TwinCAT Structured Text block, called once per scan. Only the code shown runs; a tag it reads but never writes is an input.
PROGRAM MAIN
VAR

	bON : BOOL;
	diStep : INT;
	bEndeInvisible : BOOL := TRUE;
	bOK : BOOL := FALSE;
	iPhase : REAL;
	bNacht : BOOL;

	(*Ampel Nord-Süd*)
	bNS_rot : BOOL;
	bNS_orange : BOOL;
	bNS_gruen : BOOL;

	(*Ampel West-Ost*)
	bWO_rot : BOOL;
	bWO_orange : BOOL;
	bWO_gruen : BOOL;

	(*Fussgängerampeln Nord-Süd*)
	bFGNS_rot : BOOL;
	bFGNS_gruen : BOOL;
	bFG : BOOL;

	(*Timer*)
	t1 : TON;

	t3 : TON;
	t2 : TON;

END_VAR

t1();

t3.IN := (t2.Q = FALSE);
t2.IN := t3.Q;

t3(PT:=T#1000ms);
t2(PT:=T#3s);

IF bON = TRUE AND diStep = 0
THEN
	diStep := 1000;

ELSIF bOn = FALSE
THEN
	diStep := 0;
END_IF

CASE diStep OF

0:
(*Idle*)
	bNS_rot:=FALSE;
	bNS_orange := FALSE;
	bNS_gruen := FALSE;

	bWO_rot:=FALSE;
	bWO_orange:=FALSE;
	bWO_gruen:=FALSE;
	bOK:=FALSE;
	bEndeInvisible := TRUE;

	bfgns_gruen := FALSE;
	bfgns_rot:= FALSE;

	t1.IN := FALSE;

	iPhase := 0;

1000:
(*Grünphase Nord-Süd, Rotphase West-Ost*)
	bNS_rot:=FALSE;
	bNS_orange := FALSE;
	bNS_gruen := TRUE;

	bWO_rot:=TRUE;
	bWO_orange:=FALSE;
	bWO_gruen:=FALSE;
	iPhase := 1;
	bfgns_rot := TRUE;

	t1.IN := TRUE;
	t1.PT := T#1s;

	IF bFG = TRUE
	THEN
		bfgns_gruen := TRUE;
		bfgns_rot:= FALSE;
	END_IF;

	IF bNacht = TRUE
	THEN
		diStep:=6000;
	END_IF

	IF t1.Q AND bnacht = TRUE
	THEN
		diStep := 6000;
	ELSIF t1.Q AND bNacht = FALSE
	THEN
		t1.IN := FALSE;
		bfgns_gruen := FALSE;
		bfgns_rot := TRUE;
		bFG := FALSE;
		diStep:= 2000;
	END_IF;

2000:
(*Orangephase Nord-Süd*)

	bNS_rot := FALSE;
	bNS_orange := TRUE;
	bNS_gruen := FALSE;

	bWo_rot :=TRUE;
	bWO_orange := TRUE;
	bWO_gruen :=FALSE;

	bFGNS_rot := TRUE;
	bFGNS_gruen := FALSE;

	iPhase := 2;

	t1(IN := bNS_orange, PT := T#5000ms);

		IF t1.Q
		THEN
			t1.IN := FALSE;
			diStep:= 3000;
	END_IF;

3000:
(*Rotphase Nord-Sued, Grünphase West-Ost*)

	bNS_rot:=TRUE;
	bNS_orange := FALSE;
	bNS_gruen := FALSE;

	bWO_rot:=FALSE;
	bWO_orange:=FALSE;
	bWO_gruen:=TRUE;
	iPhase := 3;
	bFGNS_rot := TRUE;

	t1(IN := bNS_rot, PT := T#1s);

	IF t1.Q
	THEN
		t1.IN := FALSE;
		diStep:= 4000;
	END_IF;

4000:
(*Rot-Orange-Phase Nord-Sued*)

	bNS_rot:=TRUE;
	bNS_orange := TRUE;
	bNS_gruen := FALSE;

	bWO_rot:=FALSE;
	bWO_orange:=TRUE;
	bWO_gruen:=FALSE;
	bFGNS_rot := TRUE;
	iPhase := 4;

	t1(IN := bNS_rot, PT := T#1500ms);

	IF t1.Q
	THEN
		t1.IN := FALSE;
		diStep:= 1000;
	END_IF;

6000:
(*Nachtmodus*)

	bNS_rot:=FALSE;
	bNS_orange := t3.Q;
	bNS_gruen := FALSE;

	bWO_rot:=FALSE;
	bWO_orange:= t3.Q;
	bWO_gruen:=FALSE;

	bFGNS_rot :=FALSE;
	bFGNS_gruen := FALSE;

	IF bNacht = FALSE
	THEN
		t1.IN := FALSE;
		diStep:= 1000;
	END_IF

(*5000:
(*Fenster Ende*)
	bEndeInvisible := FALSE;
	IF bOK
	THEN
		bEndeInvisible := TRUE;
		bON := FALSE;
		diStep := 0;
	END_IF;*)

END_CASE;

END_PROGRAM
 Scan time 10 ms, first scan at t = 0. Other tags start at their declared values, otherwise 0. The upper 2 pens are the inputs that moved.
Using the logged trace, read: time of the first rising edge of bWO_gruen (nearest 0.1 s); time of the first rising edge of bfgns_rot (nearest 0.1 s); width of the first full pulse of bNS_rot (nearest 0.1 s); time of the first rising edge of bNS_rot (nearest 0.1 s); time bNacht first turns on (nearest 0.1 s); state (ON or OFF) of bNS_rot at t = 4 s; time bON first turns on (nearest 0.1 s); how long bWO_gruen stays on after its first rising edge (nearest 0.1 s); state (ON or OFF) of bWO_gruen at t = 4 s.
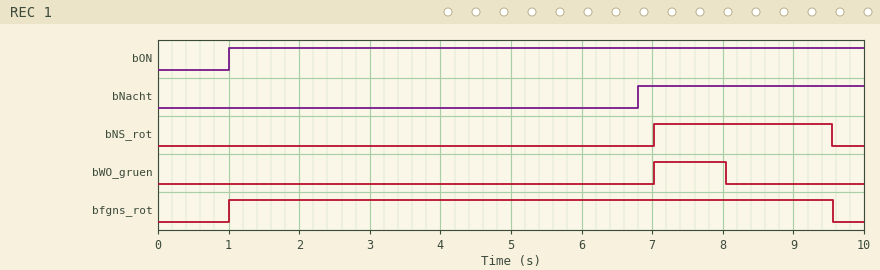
7.0 s
1.0 s
2.5 s
7.0 s
6.8 s
OFF
1.0 s
1.0 s
OFF
